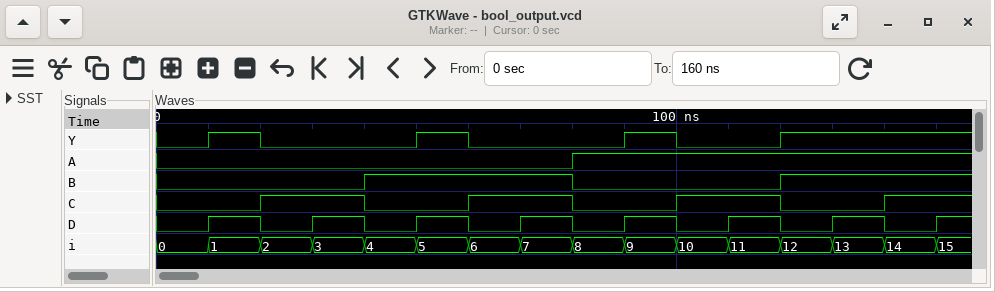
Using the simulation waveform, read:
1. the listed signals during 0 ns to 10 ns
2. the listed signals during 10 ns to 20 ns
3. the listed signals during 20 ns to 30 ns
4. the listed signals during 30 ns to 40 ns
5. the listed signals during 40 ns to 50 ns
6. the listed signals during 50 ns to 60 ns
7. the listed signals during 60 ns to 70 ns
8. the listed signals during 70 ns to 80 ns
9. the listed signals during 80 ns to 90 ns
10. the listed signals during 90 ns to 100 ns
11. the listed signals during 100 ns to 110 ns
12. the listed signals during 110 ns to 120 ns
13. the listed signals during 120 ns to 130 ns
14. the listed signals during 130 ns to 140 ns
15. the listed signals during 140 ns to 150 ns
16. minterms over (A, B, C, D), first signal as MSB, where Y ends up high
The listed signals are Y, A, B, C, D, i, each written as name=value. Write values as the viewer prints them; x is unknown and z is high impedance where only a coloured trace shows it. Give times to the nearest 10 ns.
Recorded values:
Y=0, A=0, B=0, C=0, D=0, i=0
Y=1, A=0, B=0, C=0, D=1, i=1
Y=0, A=0, B=0, C=1, D=0, i=2
Y=0, A=0, B=0, C=1, D=1, i=3
Y=0, A=0, B=1, C=0, D=0, i=4
Y=1, A=0, B=1, C=0, D=1, i=5
Y=0, A=0, B=1, C=1, D=0, i=6
Y=0, A=0, B=1, C=1, D=1, i=7
Y=0, A=1, B=0, C=0, D=0, i=8
Y=1, A=1, B=0, C=0, D=1, i=9
Y=0, A=1, B=0, C=1, D=0, i=10
Y=0, A=1, B=0, C=1, D=1, i=11
Y=1, A=1, B=1, C=0, D=0, i=12
Y=1, A=1, B=1, C=0, D=1, i=13
Y=1, A=1, B=1, C=1, D=0, i=14
1, 5, 9, 12, 13, 14, 15
